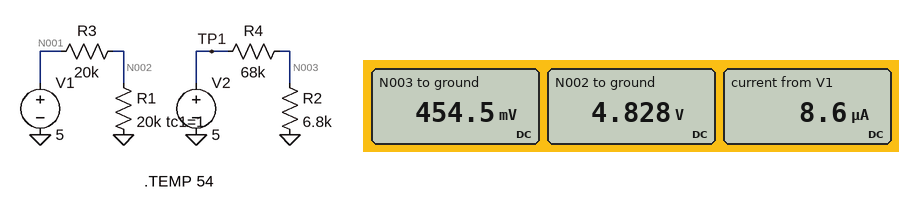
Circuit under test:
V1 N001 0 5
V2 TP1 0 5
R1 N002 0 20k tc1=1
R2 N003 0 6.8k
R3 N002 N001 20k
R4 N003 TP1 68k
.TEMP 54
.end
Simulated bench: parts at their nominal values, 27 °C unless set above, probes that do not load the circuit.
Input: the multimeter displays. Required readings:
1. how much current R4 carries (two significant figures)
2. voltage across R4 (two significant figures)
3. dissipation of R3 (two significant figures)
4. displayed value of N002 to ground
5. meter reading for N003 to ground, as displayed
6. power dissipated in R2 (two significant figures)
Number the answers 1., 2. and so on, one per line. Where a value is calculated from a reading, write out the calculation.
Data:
1. (5 V - 454.5 mV) / 68 kΩ = 67 µA
2. 5 V - 454.5 mV = 4.5 V
3. (5 V - 4.828 V)^2 / 20 kΩ = 1.5 µW
4. 4.828 V
5. 454.5 mV
6. (454.5 mV)^2 / 6.8 kΩ = 30 µW
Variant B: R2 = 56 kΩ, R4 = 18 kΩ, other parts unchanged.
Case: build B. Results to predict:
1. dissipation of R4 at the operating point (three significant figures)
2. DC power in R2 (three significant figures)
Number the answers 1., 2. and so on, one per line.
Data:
1. 82.2 µW
2. 256 µW
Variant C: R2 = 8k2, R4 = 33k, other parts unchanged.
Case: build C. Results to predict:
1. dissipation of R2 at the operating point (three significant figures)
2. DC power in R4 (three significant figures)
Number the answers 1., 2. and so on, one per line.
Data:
1. 121 µW
2. 486 µW
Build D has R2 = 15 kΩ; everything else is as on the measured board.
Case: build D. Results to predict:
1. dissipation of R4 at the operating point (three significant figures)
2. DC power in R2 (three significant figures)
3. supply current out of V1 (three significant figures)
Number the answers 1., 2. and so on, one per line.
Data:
1. 247 µW
2. 54.4 µW
3. 8.62 µA
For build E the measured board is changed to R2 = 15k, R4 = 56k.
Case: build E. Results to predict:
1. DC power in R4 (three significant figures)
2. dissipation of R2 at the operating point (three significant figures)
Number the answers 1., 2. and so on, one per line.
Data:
1. 278 µW
2. 74.4 µW
